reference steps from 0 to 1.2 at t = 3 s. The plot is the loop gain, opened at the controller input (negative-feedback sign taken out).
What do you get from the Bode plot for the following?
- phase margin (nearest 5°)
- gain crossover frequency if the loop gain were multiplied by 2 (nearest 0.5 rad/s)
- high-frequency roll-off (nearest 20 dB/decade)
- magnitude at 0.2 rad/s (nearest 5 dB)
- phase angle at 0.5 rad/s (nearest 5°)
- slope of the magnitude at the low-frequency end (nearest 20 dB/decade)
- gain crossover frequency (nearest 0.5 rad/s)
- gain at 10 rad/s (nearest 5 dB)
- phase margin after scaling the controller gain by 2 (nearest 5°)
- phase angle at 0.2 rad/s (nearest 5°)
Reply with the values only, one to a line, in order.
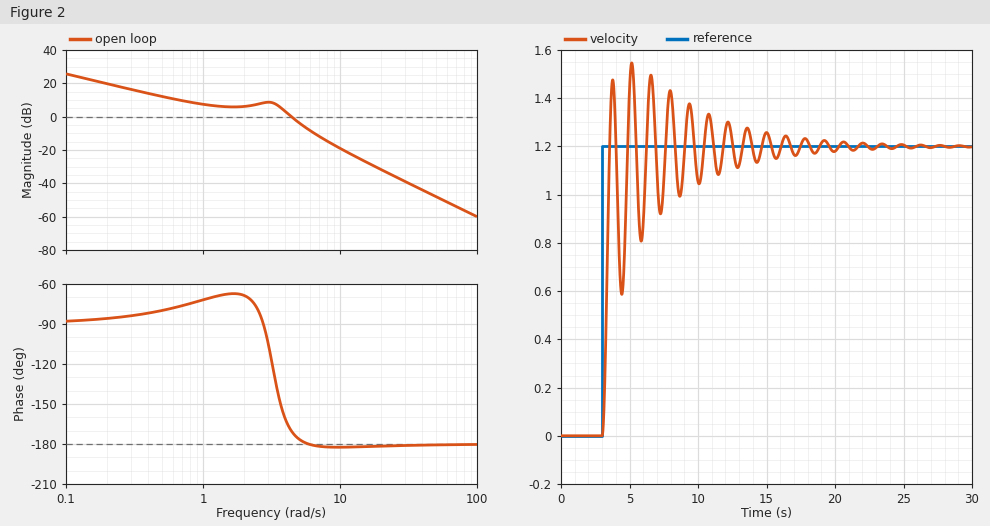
10°
5.5 rad/s
-40 dB/decade
20 dB
-80°
-20 dB/decade
4.5 rad/s
-20 dB
0°
-85°
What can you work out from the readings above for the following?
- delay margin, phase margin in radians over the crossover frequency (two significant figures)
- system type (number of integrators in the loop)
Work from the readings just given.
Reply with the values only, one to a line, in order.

0.039 s
1
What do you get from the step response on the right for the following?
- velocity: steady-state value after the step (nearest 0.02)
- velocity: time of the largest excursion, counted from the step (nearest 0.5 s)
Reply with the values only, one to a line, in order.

1.20
2.0 s
